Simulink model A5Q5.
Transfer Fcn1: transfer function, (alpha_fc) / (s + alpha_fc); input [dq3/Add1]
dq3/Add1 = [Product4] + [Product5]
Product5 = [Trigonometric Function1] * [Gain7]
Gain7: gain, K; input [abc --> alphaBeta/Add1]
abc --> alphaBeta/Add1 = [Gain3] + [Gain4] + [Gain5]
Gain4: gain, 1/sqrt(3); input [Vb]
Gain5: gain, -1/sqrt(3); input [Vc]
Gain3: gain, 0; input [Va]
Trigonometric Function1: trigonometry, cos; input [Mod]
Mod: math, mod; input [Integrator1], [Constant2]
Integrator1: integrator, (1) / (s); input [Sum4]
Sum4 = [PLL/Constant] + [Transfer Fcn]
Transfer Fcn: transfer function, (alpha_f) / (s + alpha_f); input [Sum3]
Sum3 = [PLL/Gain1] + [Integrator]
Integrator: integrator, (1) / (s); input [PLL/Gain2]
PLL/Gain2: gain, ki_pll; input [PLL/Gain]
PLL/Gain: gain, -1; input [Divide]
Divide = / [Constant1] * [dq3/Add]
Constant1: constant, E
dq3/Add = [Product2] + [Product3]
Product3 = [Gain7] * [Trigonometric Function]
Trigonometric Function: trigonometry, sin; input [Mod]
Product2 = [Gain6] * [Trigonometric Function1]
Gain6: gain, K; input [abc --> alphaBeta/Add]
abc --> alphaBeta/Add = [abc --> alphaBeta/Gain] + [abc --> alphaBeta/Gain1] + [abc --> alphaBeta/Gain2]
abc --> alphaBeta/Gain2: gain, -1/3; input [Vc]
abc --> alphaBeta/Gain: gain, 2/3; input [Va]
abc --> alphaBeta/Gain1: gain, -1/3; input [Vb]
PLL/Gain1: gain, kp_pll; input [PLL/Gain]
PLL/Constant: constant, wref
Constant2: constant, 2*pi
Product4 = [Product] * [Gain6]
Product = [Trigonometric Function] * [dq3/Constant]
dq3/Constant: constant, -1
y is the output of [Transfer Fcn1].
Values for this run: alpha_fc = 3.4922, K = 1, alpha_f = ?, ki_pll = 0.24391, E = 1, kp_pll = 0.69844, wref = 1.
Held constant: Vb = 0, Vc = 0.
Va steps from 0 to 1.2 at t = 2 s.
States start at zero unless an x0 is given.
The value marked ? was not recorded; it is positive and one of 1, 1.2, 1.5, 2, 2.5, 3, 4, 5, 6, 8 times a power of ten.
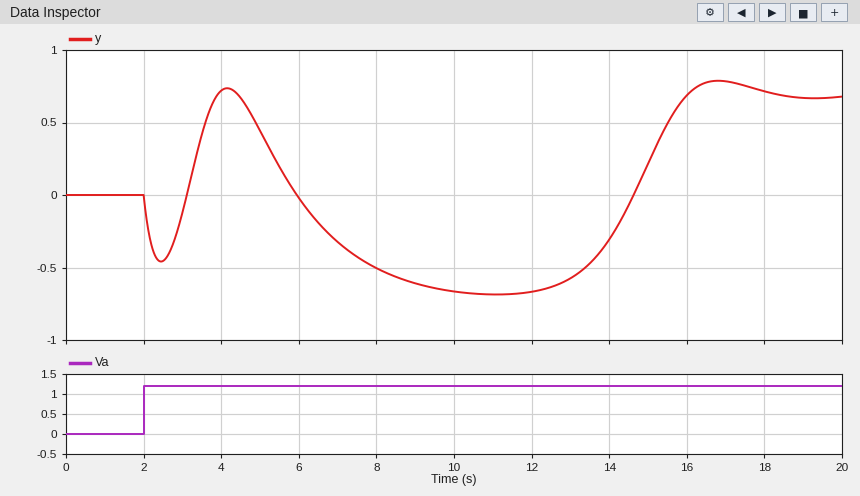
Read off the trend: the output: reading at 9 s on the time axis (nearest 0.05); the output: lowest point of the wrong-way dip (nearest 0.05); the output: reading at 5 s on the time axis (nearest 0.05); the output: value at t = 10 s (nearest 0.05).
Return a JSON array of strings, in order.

["-0.60", "-0.70", "0.45", "-0.65"]
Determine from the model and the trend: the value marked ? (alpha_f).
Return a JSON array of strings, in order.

["4"]
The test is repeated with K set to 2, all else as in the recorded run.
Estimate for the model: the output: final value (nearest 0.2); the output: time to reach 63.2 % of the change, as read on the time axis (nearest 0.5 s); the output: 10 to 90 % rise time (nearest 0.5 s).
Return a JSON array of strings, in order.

["1.6", "3.5 s", "5.0 s"]
